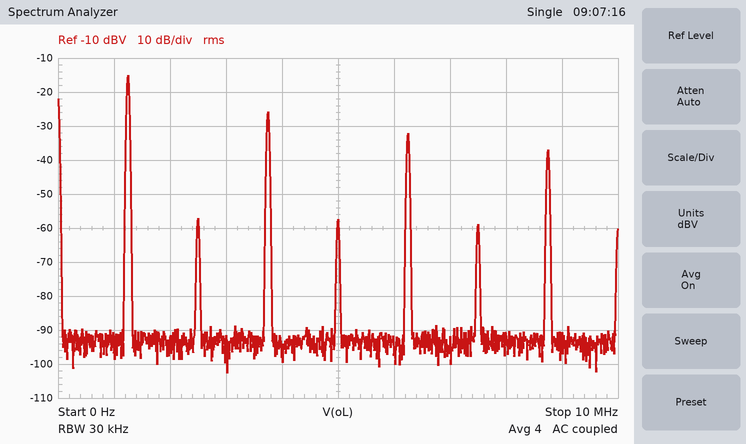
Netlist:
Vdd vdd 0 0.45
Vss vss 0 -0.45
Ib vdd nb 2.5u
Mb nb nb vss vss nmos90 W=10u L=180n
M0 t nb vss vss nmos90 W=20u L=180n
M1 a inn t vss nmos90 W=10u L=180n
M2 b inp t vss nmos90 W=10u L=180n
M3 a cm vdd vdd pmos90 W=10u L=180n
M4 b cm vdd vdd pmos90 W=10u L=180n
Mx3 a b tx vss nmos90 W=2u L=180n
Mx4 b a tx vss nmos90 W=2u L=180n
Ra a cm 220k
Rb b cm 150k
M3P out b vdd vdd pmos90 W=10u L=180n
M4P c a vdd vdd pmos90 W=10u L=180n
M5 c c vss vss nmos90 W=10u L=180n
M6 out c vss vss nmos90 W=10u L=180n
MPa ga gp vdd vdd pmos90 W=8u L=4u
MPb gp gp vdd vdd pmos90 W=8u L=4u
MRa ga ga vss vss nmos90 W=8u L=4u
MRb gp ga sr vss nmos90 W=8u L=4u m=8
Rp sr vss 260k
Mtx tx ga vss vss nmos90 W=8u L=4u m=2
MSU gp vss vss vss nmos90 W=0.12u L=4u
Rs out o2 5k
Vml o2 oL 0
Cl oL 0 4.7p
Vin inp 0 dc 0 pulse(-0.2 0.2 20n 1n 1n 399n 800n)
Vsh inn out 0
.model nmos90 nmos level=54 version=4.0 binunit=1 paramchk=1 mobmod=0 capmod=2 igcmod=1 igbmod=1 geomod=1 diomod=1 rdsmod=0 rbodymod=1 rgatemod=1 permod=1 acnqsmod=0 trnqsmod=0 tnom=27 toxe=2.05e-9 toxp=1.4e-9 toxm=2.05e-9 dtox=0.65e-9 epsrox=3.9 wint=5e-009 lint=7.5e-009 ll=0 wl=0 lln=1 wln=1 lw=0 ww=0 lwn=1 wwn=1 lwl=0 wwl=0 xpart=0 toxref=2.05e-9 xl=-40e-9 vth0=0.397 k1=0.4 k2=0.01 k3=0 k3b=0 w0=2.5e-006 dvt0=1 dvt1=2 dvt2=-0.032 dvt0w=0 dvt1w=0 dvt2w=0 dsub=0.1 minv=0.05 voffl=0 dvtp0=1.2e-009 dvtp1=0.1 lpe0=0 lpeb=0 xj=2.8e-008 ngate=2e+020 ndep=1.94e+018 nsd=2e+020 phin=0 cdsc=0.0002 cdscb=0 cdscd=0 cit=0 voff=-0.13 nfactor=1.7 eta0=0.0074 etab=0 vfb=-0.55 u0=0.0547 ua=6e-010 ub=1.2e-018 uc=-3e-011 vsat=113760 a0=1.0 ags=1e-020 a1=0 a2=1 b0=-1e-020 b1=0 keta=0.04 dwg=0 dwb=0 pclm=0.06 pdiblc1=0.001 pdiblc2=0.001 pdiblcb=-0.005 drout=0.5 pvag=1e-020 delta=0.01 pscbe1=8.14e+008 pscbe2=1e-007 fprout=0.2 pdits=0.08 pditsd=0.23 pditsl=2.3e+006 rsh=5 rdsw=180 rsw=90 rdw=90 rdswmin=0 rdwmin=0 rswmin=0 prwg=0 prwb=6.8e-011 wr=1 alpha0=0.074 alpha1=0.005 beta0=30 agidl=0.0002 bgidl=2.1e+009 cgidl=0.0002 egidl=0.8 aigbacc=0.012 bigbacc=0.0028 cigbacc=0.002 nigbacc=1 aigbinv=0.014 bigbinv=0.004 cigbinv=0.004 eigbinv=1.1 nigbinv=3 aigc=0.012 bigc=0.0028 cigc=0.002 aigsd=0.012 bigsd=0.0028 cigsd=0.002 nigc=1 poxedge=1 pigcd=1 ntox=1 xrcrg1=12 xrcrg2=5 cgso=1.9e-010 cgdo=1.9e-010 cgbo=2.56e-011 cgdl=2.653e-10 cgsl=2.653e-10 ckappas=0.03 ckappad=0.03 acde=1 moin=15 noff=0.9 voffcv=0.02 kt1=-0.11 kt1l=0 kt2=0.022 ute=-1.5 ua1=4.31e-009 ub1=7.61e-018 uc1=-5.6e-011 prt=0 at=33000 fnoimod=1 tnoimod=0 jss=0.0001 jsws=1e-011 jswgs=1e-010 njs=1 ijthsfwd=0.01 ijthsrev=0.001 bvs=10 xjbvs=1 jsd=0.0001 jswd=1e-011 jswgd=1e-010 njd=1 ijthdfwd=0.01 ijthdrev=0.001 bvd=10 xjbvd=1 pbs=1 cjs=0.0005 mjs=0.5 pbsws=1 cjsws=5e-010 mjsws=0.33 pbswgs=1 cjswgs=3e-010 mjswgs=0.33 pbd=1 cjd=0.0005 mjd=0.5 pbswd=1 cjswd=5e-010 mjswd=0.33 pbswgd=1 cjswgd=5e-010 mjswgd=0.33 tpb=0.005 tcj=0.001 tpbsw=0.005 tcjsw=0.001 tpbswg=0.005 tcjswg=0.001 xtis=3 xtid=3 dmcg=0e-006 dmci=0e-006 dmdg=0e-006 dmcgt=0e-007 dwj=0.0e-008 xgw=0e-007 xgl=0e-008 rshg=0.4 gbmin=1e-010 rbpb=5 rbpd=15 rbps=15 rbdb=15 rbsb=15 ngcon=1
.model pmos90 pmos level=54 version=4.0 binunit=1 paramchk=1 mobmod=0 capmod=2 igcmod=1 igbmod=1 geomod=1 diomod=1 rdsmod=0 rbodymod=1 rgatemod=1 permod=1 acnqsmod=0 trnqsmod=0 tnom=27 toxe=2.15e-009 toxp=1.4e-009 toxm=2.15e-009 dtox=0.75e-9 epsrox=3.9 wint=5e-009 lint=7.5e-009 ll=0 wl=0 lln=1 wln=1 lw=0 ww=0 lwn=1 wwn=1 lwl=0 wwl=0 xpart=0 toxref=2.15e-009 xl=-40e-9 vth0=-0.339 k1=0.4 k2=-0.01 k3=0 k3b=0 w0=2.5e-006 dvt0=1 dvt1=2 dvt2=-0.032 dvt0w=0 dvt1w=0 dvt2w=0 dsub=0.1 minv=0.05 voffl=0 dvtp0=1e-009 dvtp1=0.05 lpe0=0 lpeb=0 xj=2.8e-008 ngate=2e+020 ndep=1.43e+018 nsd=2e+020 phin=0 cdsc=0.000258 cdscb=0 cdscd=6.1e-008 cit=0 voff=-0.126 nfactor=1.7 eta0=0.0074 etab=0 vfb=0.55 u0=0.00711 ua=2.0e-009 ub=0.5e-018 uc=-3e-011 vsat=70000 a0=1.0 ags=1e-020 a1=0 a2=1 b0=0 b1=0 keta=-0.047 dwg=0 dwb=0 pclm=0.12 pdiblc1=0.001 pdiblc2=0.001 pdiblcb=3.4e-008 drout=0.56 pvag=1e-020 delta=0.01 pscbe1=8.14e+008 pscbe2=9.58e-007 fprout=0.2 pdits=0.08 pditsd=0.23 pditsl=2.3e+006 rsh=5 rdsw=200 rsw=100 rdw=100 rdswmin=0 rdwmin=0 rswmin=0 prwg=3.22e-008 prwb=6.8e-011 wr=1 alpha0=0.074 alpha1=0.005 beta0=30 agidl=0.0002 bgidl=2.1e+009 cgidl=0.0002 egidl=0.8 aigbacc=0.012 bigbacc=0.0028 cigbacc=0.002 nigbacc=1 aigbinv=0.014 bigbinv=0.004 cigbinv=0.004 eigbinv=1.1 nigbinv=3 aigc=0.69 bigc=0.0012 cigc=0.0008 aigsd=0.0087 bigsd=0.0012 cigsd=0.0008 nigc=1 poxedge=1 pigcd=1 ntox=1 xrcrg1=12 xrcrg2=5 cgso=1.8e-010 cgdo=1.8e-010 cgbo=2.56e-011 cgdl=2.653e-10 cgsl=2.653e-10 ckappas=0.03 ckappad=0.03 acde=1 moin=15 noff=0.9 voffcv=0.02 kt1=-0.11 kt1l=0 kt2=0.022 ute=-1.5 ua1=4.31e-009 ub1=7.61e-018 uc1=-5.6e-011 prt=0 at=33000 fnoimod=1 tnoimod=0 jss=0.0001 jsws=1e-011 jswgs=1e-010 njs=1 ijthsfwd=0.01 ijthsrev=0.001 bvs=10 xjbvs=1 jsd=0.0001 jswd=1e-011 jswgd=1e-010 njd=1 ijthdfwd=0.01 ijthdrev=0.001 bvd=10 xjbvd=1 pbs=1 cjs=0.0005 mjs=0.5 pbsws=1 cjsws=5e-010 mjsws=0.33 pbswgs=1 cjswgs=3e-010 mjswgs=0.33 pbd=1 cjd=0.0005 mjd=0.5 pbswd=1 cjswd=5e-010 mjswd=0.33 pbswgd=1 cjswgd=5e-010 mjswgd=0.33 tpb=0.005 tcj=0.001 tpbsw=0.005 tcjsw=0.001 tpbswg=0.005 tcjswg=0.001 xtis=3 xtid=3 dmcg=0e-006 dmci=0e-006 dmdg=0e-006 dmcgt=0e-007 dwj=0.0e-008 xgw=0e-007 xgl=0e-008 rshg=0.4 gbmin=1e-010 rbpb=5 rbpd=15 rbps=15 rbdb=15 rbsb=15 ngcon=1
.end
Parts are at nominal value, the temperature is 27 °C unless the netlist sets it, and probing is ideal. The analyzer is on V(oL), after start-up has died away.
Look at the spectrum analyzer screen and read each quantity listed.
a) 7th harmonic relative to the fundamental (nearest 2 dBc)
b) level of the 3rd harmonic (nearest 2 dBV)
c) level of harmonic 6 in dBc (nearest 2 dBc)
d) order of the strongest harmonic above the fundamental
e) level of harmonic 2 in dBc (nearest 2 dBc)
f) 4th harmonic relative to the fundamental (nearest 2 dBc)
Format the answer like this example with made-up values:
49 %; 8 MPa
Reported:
-22 dBc; -26 dBV; -44 dBc; 3; -42 dBc; -42 dBc
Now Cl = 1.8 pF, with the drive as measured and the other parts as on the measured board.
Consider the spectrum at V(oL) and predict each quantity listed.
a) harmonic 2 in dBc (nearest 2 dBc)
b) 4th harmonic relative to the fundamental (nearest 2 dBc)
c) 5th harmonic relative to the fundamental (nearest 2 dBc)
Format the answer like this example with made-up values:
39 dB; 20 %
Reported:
-40 dBc; -40 dBc; -14 dBc
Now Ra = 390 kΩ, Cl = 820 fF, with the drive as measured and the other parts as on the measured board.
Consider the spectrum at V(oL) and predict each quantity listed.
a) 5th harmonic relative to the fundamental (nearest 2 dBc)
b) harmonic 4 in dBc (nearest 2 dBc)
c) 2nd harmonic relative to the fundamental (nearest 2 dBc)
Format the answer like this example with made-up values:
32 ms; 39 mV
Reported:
-14 dBc; -44 dBc; -44 dBc
